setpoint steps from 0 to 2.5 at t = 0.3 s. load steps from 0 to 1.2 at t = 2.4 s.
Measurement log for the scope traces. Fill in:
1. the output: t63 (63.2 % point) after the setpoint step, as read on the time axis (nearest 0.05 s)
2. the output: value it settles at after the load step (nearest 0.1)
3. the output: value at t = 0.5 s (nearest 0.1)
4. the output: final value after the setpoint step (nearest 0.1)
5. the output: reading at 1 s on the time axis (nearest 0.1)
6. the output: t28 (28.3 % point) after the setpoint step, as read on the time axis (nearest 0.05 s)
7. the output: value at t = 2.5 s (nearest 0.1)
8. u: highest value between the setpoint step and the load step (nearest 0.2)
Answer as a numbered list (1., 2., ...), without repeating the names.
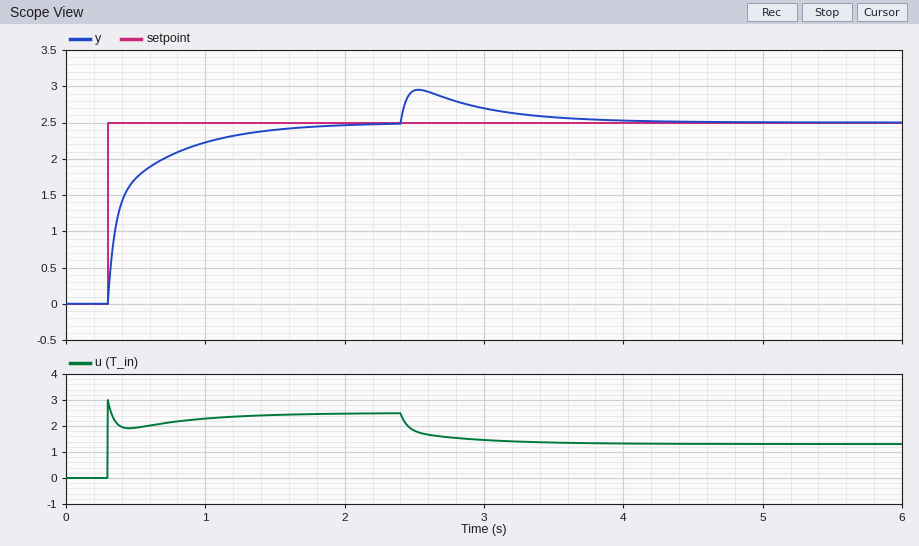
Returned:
1. 0.45 s
2. 2.5
3. 1.7
4. 2.5
5. 2.2
6. 0.35 s
7. 2.9
8. 3.0
